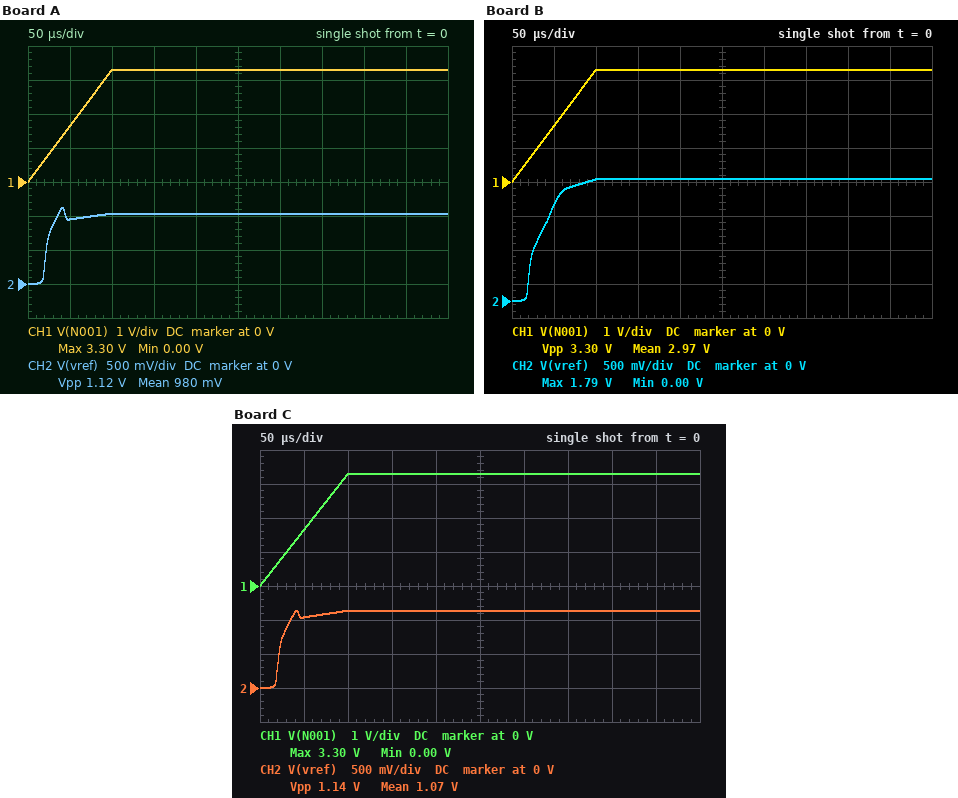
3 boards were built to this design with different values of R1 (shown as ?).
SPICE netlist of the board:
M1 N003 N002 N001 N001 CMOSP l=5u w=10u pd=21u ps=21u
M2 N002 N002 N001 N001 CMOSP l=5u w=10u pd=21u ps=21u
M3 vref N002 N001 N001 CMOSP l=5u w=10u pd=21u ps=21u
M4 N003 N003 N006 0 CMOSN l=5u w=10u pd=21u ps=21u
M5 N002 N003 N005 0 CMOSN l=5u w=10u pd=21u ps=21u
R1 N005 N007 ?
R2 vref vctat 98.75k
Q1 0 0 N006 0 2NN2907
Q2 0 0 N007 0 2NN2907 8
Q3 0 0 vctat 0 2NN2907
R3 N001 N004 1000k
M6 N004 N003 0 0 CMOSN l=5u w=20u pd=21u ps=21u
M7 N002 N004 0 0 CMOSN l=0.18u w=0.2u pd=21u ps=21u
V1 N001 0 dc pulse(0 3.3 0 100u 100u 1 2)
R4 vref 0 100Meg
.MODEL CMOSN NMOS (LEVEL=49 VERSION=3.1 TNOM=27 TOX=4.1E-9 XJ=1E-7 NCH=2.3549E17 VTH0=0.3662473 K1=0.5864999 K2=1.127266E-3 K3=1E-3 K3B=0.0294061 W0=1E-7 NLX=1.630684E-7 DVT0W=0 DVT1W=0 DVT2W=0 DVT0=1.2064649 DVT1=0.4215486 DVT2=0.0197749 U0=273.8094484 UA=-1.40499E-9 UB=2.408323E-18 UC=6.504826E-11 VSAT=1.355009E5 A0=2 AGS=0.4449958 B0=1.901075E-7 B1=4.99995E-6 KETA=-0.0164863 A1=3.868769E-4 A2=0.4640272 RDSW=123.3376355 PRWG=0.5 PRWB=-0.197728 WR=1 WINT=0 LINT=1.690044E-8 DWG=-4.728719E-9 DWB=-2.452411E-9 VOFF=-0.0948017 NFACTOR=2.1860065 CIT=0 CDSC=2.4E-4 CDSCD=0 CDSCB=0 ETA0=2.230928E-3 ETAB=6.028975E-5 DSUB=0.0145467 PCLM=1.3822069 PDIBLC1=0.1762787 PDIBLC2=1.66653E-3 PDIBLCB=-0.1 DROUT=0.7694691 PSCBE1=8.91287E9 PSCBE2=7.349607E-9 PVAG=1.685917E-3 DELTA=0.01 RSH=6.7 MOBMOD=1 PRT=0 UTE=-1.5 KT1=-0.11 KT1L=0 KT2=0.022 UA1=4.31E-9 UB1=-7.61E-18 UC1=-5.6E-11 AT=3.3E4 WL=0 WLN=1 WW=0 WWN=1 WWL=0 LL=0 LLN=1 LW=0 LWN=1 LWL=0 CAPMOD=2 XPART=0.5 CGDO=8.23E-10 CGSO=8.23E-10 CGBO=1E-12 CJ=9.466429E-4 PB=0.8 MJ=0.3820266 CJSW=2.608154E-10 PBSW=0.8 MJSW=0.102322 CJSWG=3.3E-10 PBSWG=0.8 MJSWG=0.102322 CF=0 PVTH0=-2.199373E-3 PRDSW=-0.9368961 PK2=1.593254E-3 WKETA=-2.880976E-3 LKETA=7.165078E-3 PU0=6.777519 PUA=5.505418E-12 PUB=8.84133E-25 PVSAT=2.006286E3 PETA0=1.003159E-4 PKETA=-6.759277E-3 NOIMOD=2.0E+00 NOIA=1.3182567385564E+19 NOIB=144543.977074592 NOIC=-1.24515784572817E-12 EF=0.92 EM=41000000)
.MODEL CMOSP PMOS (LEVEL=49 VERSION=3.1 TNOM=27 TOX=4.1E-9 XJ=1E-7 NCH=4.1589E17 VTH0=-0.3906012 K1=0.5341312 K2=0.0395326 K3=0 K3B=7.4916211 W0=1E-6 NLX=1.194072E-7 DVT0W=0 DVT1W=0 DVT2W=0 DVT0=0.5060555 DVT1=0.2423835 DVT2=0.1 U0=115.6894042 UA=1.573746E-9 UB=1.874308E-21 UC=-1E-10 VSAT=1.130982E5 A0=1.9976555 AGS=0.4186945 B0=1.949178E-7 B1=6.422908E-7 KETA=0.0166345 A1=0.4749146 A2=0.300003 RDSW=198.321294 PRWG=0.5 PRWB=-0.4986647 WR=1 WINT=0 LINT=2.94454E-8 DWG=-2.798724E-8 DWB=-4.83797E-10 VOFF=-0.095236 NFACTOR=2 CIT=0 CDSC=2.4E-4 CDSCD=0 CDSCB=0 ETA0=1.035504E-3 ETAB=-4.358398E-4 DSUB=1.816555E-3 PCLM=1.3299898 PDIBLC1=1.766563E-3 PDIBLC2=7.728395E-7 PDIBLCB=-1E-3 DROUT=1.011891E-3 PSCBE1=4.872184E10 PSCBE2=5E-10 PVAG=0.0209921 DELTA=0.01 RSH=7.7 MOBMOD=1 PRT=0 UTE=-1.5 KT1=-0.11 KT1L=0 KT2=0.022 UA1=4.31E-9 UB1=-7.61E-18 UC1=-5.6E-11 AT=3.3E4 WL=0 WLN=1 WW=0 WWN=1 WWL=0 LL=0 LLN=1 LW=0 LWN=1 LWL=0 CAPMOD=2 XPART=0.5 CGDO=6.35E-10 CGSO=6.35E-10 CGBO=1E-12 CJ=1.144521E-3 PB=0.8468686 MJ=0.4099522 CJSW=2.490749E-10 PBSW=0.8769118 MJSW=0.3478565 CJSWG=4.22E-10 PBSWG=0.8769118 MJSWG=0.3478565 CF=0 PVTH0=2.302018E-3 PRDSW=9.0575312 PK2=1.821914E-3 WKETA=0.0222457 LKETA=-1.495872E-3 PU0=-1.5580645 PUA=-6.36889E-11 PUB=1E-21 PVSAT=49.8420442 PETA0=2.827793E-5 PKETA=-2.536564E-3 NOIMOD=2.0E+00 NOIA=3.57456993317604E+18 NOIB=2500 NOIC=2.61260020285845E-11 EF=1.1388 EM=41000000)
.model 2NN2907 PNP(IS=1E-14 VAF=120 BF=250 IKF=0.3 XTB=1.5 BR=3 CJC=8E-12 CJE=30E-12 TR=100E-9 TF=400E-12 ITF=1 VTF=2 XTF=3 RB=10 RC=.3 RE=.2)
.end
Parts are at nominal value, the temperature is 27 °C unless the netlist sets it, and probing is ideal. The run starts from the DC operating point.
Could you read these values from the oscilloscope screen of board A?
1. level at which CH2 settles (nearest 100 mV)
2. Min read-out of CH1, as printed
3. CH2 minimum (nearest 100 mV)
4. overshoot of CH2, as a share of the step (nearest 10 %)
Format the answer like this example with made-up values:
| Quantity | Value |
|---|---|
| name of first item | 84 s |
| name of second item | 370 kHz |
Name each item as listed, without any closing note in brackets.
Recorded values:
| Quantity | Value |
|---|---|
| level at which CH2 settles | 1.0 V |
| Min read-out of CH1, as printed | 0.00 V |
| CH2 minimum | 0 V |
| overshoot of CH2, as a share of the step | 10 % |
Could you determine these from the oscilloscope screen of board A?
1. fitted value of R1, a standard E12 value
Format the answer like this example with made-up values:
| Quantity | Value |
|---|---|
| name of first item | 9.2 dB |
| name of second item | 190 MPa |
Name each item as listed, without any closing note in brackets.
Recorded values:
| Quantity | Value |
|---|---|
| fitted value of R1, a standard E12 value | 12 kΩ |
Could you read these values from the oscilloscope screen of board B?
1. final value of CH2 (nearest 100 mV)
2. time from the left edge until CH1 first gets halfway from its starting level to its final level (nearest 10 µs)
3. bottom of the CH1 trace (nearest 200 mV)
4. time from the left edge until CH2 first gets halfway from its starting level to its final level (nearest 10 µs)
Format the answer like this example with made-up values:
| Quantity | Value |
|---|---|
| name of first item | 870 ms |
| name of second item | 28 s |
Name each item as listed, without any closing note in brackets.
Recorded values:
| Quantity | Value |
|---|---|
| final value of CH2 | 1.8 V |
| time from the left edge until CH1 first gets halfway from its starting level to its final level | 50 µs |
| bottom of the CH1 trace | 0 V |
| time from the left edge until CH2 first gets halfway from its starting level to its final level | 30 µs |
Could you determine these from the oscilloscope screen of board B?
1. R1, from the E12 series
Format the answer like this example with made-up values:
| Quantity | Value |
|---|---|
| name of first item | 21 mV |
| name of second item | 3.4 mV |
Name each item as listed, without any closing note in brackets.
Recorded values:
| Quantity | Value |
|---|---|
| R1, from the E12 series | 4.7 kΩ |
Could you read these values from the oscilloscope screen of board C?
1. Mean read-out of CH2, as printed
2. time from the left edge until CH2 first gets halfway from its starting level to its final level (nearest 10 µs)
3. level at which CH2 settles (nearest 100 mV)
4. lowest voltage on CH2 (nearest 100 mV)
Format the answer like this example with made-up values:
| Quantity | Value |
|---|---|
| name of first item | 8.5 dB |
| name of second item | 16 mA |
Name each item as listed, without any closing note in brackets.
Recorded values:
| Quantity | Value |
|---|---|
| Mean read-out of CH2, as printed | 1.07 V |
| time from the left edge until CH2 first gets halfway from its starting level to its final level | 20 µs |
| level at which CH2 settles | 1.1 V |
| lowest voltage on CH2 | 0 V |
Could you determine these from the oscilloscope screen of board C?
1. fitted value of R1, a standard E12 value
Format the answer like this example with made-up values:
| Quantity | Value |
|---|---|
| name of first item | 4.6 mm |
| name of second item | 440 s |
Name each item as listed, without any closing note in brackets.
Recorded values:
| Quantity | Value |
|---|---|
| fitted value of R1, a standard E12 value | 10 kΩ |
